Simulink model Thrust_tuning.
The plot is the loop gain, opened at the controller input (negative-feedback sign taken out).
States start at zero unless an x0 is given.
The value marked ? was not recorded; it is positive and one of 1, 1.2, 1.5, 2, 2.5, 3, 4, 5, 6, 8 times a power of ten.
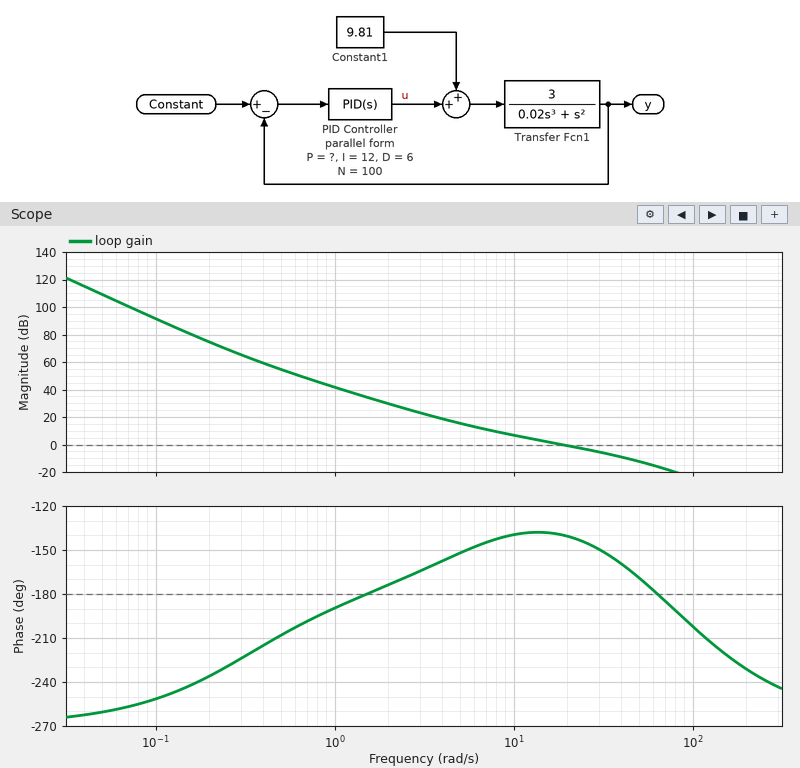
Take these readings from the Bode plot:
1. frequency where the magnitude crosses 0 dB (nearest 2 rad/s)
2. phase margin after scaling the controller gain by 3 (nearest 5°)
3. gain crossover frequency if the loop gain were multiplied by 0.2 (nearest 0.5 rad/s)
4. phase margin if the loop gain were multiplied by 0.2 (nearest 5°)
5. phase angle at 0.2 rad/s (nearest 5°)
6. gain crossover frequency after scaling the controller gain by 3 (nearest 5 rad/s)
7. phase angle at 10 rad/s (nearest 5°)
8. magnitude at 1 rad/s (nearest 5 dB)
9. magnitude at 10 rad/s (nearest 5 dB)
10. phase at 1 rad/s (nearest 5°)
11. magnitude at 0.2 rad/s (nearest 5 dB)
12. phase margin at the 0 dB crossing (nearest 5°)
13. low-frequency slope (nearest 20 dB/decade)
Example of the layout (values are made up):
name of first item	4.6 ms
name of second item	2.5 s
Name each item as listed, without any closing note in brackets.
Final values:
frequency where the magnitude crosses 0 dB	18 rad/s
phase margin after scaling the controller gain by 3	20°
gain crossover frequency if the loop gain were multiplied by 0.2	5.5 rad/s
phase margin if the loop gain were multiplied by 0.2	30°
phase angle at 0.2 rad/s	-235°
gain crossover frequency after scaling the controller gain by 3	40 rad/s
phase angle at 10 rad/s	-140°
magnitude at 1 rad/s	40 dB
magnitude at 10 rad/s	5 dB
phase at 1 rad/s	-190°
magnitude at 0.2 rad/s	75 dB
phase margin at the 0 dB crossing	40°
low-frequency slope	-60 dB/decade
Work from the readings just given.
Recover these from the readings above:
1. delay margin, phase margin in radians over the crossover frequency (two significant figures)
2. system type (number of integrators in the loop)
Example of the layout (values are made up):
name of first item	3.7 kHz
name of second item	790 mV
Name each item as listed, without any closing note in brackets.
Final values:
delay margin, phase margin in radians over the crossover frequency	0.039 s
system type	3
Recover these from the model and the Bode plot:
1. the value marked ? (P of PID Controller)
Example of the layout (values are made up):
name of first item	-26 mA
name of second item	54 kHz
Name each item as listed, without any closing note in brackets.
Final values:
the value marked ?	40
